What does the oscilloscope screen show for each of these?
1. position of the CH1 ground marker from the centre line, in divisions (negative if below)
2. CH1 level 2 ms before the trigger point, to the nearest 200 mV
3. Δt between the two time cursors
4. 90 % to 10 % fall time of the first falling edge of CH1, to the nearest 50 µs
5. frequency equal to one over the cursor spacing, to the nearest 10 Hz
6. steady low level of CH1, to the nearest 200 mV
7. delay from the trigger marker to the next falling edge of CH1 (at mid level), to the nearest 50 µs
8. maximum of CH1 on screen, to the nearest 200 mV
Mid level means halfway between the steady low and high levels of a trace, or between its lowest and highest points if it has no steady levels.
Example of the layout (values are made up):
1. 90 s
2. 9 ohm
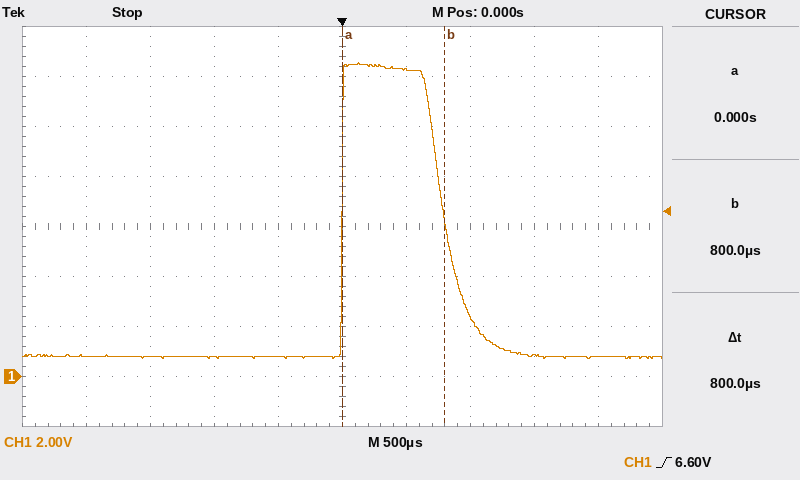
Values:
1. -3.0 div
2. 800 mV
3. 800 µs
4. 400 µs
5. 1.25 kHz
6. 800 mV
7. 800 µs
8. 12.6 V
